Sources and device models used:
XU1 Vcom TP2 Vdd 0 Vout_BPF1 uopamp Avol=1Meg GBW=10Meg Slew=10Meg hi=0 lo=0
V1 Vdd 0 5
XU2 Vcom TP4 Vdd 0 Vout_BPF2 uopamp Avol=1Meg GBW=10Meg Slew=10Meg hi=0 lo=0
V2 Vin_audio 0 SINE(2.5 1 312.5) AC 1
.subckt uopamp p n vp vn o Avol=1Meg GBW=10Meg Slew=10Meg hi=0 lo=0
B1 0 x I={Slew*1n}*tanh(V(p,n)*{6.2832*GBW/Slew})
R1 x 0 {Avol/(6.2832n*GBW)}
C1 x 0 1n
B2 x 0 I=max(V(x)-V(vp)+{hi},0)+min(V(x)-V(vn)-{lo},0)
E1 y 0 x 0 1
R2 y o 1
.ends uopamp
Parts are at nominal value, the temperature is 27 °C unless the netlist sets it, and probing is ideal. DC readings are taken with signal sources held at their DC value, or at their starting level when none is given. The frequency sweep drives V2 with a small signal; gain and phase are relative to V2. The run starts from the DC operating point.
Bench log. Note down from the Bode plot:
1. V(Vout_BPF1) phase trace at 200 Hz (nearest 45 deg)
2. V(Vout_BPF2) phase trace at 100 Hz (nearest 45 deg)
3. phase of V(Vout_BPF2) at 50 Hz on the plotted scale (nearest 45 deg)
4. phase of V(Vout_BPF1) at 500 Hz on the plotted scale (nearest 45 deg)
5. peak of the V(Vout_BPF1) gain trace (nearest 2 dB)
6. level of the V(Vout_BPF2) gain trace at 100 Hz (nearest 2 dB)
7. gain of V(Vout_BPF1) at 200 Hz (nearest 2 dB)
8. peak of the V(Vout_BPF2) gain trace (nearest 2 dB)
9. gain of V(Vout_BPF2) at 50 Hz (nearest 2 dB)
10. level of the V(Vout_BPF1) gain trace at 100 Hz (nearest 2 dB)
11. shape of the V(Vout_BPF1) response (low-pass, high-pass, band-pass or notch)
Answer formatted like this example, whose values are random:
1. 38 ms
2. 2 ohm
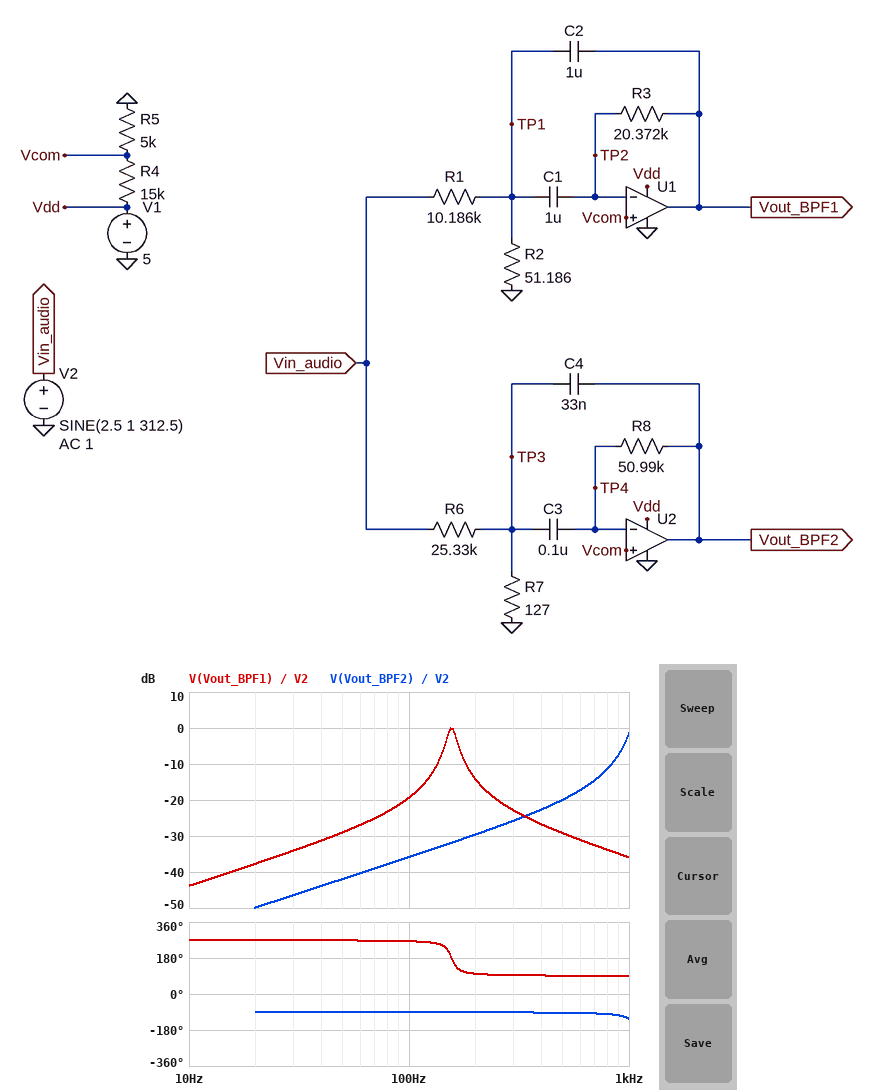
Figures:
1. 90 deg
2. -90 deg
3. -90 deg
4. 90 deg
5. 0 dB
6. -36 dB
7. -14 dB
8. -2 dB
9. -42 dB
10. -20 dB
11. band-pass
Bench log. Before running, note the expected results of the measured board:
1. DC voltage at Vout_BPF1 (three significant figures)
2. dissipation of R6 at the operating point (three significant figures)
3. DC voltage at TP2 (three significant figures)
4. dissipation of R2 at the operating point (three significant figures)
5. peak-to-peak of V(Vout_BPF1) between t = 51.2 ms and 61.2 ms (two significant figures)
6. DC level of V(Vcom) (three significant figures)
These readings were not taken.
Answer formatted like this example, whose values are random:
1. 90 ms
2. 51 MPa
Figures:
1. 1.25 V
2. 244 µW
3. 1.25 V
4. 3.05 µW
5. 140 mV
6. 1.25 V
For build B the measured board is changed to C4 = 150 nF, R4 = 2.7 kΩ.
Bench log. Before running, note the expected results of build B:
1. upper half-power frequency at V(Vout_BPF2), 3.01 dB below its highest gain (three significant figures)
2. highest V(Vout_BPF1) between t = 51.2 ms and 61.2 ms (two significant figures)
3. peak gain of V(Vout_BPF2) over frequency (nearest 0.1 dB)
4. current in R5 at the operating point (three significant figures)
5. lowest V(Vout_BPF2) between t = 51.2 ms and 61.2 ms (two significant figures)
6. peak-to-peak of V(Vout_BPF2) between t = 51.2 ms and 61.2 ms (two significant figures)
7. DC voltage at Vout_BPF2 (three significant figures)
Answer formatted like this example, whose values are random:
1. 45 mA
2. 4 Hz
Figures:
1. 538 Hz
2. 3.3 V
3. -1.9 dB
4. 649 µA
5. 3.2 V
6. 160 mV
7. 3.25 V
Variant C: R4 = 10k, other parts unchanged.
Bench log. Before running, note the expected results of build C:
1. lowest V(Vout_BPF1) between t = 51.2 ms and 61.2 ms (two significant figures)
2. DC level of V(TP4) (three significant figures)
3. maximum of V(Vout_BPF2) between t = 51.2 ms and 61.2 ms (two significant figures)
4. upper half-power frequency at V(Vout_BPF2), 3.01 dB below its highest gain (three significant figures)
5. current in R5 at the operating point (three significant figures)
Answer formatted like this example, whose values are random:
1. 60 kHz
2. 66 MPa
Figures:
1. 1.6 V
2. 1.67 V
3. 1.7 V
4. 1.15 kHz
5. 333 µA
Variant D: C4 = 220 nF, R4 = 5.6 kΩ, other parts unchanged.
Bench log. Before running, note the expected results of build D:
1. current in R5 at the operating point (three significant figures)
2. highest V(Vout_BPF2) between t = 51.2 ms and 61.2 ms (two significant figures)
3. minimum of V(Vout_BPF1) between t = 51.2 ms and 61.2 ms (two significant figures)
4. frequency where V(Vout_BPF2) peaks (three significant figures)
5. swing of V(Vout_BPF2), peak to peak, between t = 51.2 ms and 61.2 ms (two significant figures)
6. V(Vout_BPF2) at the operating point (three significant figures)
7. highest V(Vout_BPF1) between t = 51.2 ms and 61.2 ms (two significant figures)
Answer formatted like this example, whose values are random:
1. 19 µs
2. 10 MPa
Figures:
1. 472 µA
2. 2.5 V
3. 2.3 V
4. 423 Hz
5. 220 mV
6. 2.36 V
7. 2.4 V
